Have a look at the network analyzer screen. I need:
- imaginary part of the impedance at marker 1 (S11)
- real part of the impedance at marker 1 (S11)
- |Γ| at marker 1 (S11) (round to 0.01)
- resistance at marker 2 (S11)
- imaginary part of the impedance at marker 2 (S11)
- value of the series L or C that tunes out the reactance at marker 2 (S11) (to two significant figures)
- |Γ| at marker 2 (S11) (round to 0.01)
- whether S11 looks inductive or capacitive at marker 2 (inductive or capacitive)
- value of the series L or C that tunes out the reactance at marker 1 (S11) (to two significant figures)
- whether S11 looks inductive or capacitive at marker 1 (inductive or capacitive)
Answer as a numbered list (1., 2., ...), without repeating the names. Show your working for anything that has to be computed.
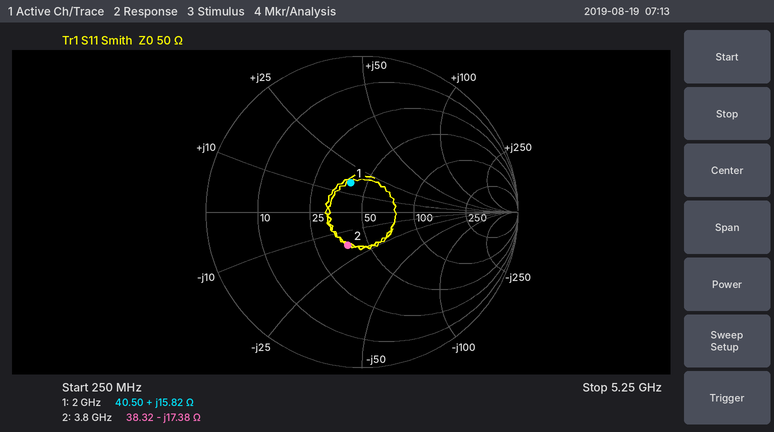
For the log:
1. +15.82 Ω
2. 40.50 Ω
3. 0.20
4. 38.32 Ω
5. -17.38 Ω
6. L = 17.38 Ω/(2π × 3.8 GHz) ≈ 728 pH, so 730 pH to two significant figures
7. 0.23
8. capacitive
9. C = 1/(2π × 2 GHz × 15.82 Ω) ≈ 5.0 pF
10. inductive
